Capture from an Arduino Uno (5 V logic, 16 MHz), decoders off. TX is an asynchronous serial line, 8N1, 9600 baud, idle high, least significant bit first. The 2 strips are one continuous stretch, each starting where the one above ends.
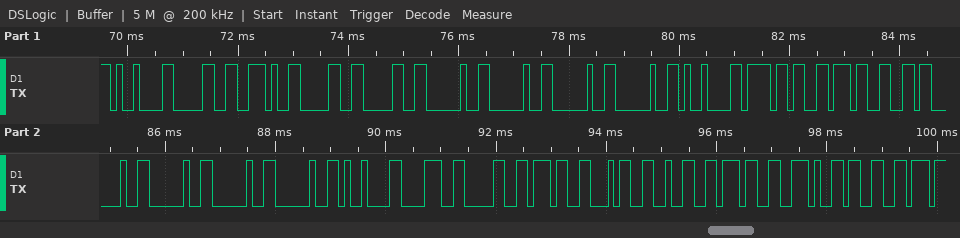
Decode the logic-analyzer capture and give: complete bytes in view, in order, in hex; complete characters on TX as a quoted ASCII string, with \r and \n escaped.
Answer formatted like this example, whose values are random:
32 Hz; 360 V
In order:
09 30 2E 30 30 20 20 20 20 09 6F 76 66 20 20 20 20 09 38 30 37 34 32 37 2E 33; "\t0.00    \tovf    \t807427.3"
